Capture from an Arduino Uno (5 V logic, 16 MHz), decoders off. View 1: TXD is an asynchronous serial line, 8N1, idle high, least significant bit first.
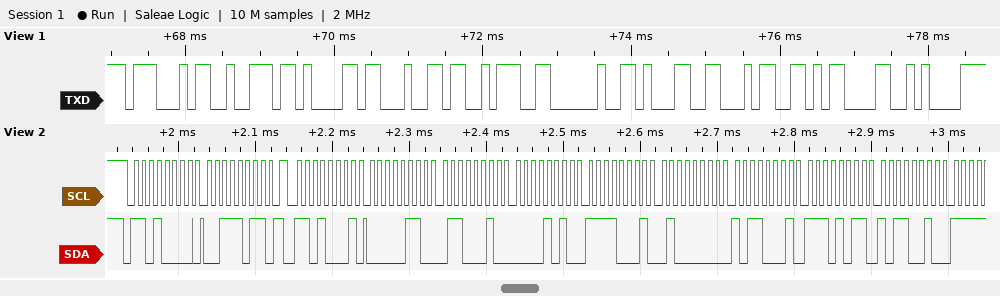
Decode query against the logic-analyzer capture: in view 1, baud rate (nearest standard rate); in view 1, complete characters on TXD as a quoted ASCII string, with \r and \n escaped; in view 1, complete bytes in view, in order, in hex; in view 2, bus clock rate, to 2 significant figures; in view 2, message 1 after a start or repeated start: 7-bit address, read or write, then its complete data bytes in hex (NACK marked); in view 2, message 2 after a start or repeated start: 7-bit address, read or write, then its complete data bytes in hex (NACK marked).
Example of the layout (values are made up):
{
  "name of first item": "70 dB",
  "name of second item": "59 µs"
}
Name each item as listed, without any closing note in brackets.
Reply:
{
  "in view 1, baud rate": "9600 baud",
  "in view 1, complete characters on TXD as a quoted ASCII string, with \\r and \\n escaped": "\"Grad: 14\\r\\n\"",
  "in view 1, complete bytes in view, in order, in hex": "47 72 61 64 3A 20 31 34 0D 0A",
  "in view 2, bus clock rate, to 2 significant figures": "100 kHz",
  "in view 2, message 1 after a start or repeated start: 7-bit address, read or write, then its complete data bytes in hex": "0x68 write: 3B",
  "in view 2, message 2 after a start or repeated start: 7-bit address, read or write, then its complete data bytes in hex": "0x68 read: 06 62 0A F1 40 B1 EB B2"
}
